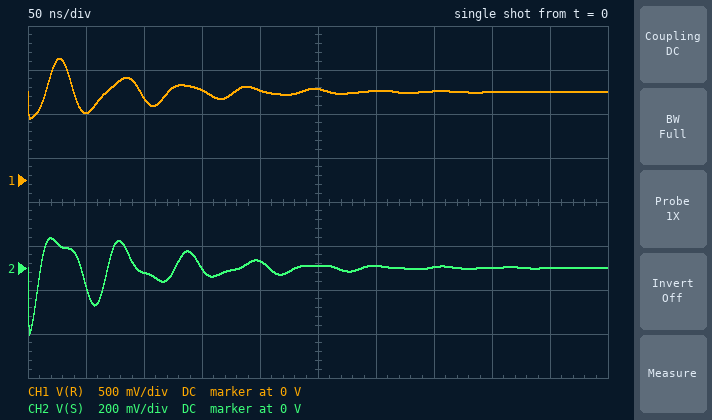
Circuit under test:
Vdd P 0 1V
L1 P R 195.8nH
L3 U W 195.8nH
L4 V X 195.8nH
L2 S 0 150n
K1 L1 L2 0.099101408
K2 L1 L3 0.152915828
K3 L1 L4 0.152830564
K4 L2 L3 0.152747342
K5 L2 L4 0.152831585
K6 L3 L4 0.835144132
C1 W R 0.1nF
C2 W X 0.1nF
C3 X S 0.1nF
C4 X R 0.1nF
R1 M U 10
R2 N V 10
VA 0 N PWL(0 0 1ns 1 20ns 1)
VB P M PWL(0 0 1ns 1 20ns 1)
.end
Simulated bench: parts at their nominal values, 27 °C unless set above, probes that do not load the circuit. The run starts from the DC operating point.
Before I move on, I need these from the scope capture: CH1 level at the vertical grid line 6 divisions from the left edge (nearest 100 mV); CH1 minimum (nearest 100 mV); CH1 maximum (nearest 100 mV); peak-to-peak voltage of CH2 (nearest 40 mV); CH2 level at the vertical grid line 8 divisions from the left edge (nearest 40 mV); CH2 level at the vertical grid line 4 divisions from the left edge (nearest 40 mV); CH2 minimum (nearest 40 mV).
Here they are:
1.0 V
700 mV
1.4 V
440 mV
0 V
40 mV
-320 mV
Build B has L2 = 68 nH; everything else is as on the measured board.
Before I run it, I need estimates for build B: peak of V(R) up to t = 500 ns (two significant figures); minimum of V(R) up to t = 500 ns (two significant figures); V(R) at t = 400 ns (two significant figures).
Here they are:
1.5 V
680 mV
1.0 V
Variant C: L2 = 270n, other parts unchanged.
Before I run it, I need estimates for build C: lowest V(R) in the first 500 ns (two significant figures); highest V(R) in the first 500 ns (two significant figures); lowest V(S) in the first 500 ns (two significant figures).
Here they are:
630 mV
1.3 V
-370 mV
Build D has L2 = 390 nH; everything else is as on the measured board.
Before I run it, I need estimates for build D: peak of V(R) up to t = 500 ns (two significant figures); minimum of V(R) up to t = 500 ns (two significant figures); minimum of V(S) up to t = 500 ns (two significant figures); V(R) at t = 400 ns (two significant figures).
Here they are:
1.3 V
600 mV
-530 mV
970 mV
